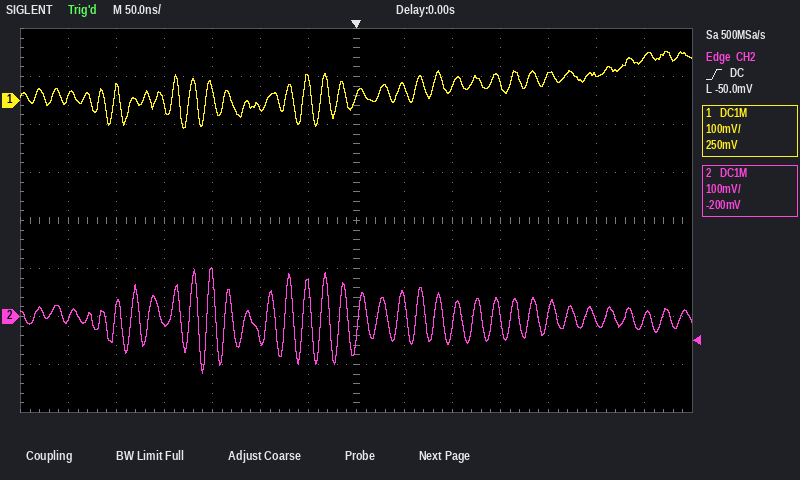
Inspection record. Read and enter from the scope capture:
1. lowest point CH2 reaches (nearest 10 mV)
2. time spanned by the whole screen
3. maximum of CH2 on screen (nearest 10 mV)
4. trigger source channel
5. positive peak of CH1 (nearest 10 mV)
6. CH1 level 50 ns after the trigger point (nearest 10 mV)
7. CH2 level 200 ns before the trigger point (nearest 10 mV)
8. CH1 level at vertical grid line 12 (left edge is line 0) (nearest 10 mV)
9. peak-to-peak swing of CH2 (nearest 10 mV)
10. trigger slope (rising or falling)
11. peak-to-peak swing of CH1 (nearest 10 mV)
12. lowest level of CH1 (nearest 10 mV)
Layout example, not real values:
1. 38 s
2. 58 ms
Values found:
1. -120 mV
2. 700 ns
3. 100 mV
4. CH2
5. 100 mV
6. 30 mV
7. -20 mV
8. 50 mV
9. 220 mV
10. rising
11. 160 mV
12. -60 mV
